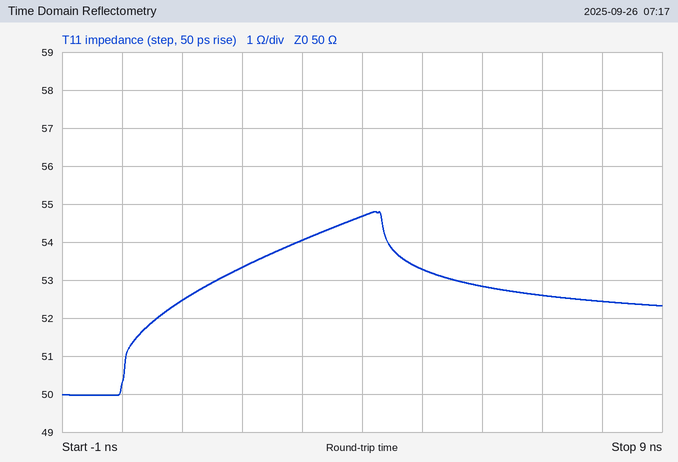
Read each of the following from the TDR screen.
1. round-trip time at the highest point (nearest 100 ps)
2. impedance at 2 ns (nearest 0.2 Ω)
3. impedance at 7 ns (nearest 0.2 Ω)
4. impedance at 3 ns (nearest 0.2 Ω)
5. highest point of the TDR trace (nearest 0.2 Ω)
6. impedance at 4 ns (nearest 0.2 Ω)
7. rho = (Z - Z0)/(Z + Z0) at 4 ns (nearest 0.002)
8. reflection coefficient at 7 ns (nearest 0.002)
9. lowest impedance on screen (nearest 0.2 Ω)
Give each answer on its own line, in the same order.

4.2 ns
53.4 Ω
52.6 Ω
54.0 Ω
54.8 Ω
54.6 Ω
+0.044
+0.026
50.0 Ω
